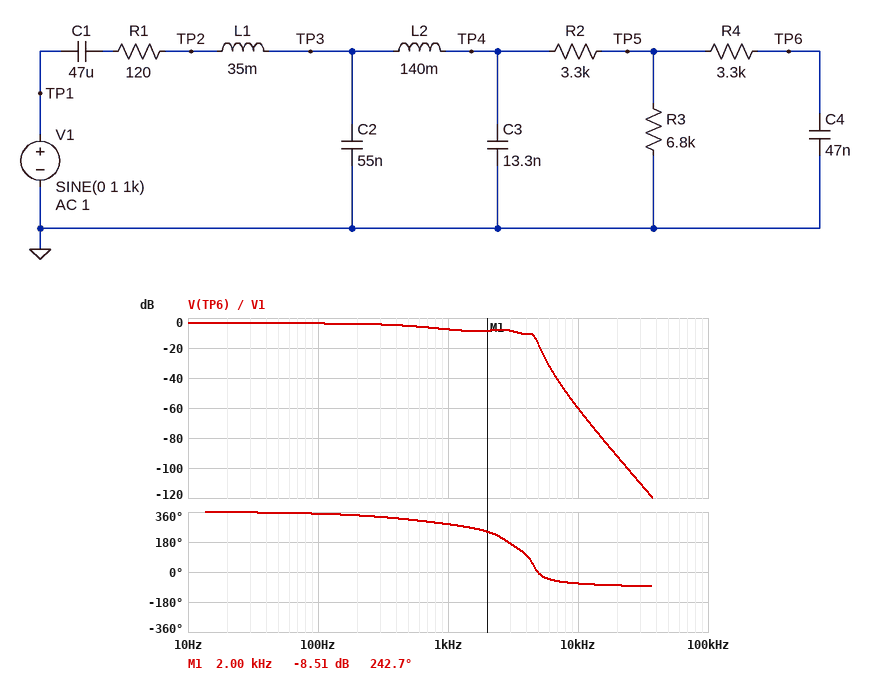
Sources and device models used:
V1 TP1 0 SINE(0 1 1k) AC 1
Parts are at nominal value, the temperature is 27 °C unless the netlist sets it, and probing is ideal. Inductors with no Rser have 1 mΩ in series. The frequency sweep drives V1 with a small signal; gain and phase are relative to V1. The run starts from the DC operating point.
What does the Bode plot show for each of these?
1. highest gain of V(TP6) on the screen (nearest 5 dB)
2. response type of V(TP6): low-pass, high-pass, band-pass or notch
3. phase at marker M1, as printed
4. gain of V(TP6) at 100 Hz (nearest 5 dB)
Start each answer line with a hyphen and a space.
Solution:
- -5 dB
- low-pass
- 242.7 deg
- -5 dB
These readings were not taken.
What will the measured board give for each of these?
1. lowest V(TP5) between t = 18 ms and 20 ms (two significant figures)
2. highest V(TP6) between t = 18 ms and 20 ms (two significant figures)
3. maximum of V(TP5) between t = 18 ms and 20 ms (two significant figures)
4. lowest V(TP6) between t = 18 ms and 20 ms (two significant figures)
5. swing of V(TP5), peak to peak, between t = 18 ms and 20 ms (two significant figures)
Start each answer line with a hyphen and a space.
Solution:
- -580 mV
- 420 mV
- 580 mV
- -420 mV
- 1.2 V
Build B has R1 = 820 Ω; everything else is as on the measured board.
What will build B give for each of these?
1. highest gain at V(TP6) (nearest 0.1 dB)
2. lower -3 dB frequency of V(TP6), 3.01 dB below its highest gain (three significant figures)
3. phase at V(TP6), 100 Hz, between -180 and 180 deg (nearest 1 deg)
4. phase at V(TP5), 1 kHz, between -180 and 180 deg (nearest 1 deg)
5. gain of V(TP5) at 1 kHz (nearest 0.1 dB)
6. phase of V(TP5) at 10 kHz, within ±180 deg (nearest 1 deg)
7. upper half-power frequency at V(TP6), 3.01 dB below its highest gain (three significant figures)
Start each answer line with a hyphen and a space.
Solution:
- -4.1 dB
- 309 mHz
- -12 deg
- -44 deg
- -6.4 dB
- 35 deg
- 634 Hz
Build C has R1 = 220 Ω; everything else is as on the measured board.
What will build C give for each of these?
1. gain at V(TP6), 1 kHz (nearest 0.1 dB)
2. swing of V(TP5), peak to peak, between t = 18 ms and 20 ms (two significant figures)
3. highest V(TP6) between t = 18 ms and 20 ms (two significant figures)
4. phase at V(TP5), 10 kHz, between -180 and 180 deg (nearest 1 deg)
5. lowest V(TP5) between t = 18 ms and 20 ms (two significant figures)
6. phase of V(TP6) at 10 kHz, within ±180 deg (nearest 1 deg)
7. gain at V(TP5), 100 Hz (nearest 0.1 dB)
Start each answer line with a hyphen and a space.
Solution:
- -7.8 dB
- 1.1 V
- 410 mV
- 18 deg
- -570 mV
- -66 deg
- -3.7 dB
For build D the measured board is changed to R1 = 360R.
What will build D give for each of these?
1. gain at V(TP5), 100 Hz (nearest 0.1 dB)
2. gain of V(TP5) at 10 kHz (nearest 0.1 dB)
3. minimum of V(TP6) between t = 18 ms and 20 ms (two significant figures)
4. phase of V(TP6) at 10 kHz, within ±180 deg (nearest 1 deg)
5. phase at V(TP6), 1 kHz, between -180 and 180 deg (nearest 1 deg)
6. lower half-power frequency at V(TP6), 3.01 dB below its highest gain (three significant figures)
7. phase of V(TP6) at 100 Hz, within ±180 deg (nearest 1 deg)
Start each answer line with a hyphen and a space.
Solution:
- -3.8 dB
- -40.4 dB
- -390 mV
- -62 deg
- -79 deg
- 323 mHz
- -11 deg
